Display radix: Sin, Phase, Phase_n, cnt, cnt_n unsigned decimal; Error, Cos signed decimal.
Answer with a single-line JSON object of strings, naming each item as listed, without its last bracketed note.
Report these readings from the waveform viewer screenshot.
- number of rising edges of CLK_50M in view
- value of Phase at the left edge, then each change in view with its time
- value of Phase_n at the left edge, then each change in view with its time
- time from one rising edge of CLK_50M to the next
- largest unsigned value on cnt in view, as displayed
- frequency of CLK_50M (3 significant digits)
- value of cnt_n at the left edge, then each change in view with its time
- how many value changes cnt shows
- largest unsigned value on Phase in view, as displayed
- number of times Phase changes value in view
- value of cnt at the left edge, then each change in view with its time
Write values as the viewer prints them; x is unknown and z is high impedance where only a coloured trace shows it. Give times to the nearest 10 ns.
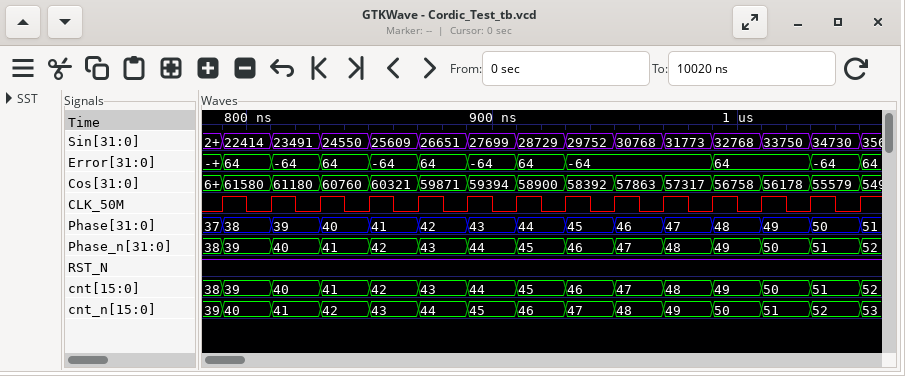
{"number of rising edges of CLK_50M in view": "14", "value of Phase at the left edge, then each change in view with its time": "37, 38 at 790 ns, 39 at 810 ns, 40 at 830 ns, 41 at 850 ns, 42 at 870 ns, 43 at 890 ns, 44 at 910 ns, 45 at 930 ns, 46 at 950 ns, 47 at 970 ns, 48 at 990 ns, 49 at 1010 ns, 50 at 1030 ns, 51 at 1050 ns", "value of Phase_n at the left edge, then each change in view with its time": "38, 39 at 790 ns, 40 at 810 ns, 41 at 830 ns, 42 at 850 ns, 43 at 870 ns, 44 at 890 ns, 45 at 910 ns, 46 at 930 ns, 47 at 950 ns, 48 at 970 ns, 49 at 990 ns, 50 at 1010 ns, 51 at 1030 ns, 52 at 1050 ns", "time from one rising edge of CLK_50M to the next": "20 ns", "largest unsigned value on cnt in view, as displayed": "52", "frequency of CLK_50M": "50.0 MHz", "value of cnt_n at the left edge, then each change in view with its time": "39, 40 at 790 ns, 41 at 810 ns, 42 at 830 ns, 43 at 850 ns, 44 at 870 ns, 45 at 890 ns, 46 at 910 ns, 47 at 930 ns, 48 at 950 ns, 49 at 970 ns, 50 at 990 ns, 51 at 1010 ns, 52 at 1030 ns, 53 at 1050 ns", "how many value changes cnt shows": "14", "largest unsigned value on Phase in view, as displayed": "51", "number of times Phase changes value in view": "14", "value of cnt at the left edge, then each change in view with its time": "38, 39 at 790 ns, 40 at 810 ns, 41 at 830 ns, 42 at 850 ns, 43 at 870 ns, 44 at 890 ns, 45 at 910 ns, 46 at 930 ns, 47 at 950 ns, 48 at 970 ns, 49 at 990 ns, 50 at 1010 ns, 51 at 1030 ns, 52 at 1050 ns"}
